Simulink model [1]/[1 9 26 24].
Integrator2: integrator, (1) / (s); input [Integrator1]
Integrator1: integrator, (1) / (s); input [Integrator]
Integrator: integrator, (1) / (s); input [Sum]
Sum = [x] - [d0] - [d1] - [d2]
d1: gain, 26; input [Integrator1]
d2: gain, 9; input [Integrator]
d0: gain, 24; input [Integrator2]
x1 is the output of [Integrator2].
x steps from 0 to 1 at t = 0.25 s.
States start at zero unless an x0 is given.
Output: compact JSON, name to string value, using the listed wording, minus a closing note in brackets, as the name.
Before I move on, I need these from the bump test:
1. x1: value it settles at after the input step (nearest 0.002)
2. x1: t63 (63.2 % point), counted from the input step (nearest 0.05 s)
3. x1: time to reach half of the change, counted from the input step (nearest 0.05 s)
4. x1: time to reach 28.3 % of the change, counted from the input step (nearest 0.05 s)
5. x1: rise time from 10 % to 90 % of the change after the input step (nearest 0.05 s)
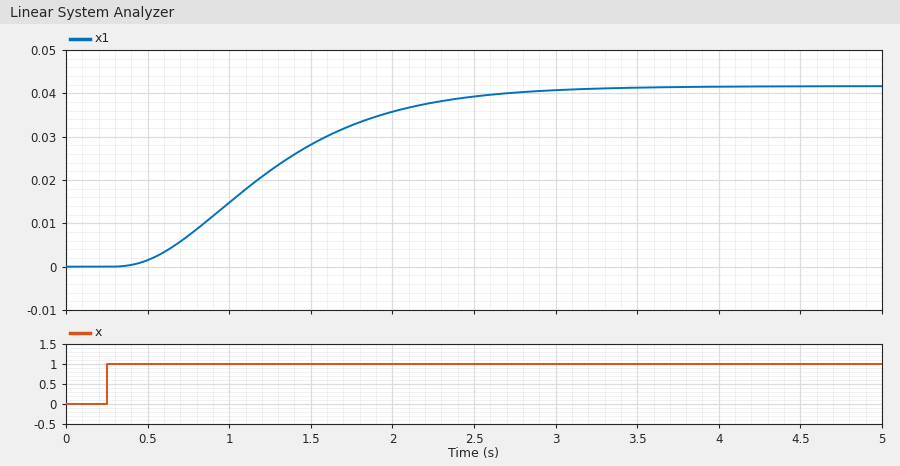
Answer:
{"x1: value it settles at after the input step": "0.042", "x1: t63 (63.2 % point), counted from the input step": "1.15 s", "x1: time to reach half of the change, counted from the input step": "0.95 s", "x1: time to reach 28.3 % of the change, counted from the input step": "0.65 s", "x1: rise time from 10 % to 90 % of the change after the input step": "1.55 s"}
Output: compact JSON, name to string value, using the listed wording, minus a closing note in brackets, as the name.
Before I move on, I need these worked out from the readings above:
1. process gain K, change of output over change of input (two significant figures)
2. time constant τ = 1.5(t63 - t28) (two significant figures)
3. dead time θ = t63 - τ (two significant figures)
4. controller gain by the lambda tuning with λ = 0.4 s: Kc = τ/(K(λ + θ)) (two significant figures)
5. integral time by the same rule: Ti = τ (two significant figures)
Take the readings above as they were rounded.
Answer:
{"process gain K, change of output over change of input": "0.042", "time constant τ = 1.5(t63 - t28)": "0.75 s", "dead time θ = t63 - τ": "0.40 s", "controller gain by the lambda tuning with λ = 0.4 s: Kc = τ/(K(λ + θ))": "22", "integral time by the same rule: Ti = τ": "0.75 s"}
